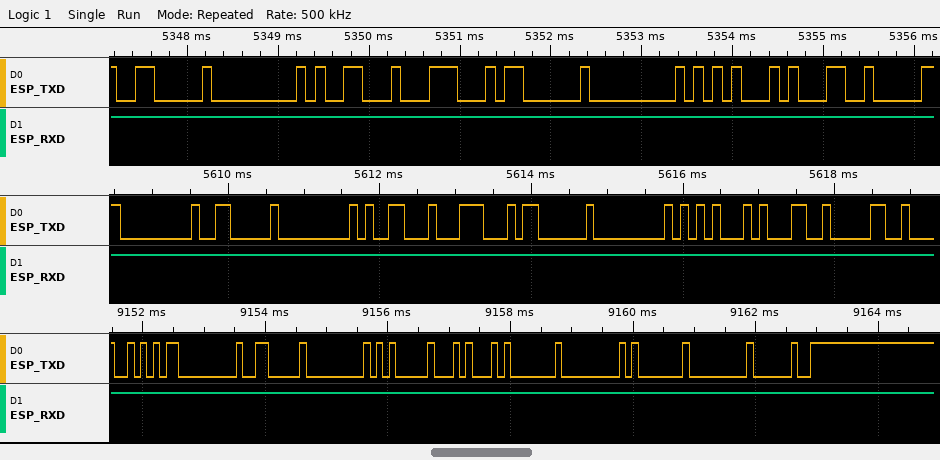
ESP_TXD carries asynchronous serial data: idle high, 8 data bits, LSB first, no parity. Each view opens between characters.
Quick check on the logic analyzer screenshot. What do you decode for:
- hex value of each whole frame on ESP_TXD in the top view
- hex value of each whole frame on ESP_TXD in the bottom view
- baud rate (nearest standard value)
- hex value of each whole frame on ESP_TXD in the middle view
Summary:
06, 00, 19, 1C, 03, 00, 15, 31
AA, 00, 06, 00, 05, 14, 01, 00, 01, 00, 20
9600 baud
00, 06, 00, 19, 1C, 03, 00, 15, 31, 30
